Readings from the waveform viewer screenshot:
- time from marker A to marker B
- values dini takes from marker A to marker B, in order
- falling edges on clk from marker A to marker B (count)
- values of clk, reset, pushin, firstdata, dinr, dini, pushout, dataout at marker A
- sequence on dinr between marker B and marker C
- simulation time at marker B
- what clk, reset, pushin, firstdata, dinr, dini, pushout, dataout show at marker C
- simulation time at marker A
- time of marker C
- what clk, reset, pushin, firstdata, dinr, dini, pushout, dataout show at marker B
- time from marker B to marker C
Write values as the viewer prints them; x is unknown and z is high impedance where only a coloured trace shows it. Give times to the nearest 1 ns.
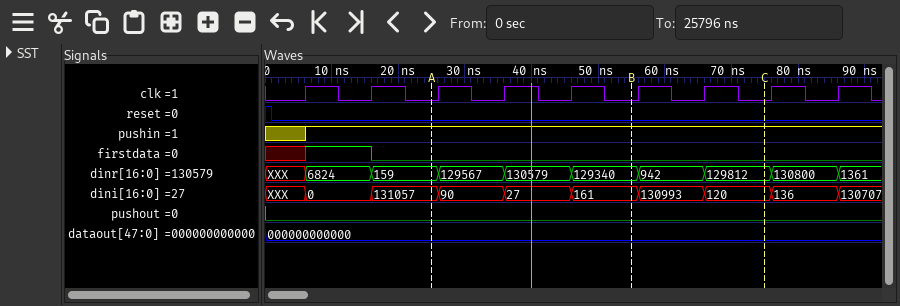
30 ns
131057, 90, 27, 161
3
clk=0, reset=0, pushin=1, firstdata=0, dinr=159, dini=131057, pushout=0, dataout=000000000000
129340, 942, 129812
55 ns
clk=0, reset=0, pushin=1, firstdata=0, dinr=129812, dini=120, pushout=0, dataout=000000000000
25 ns
75 ns
clk=0, reset=0, pushin=1, firstdata=0, dinr=129340, dini=161, pushout=0, dataout=000000000000
20 ns
